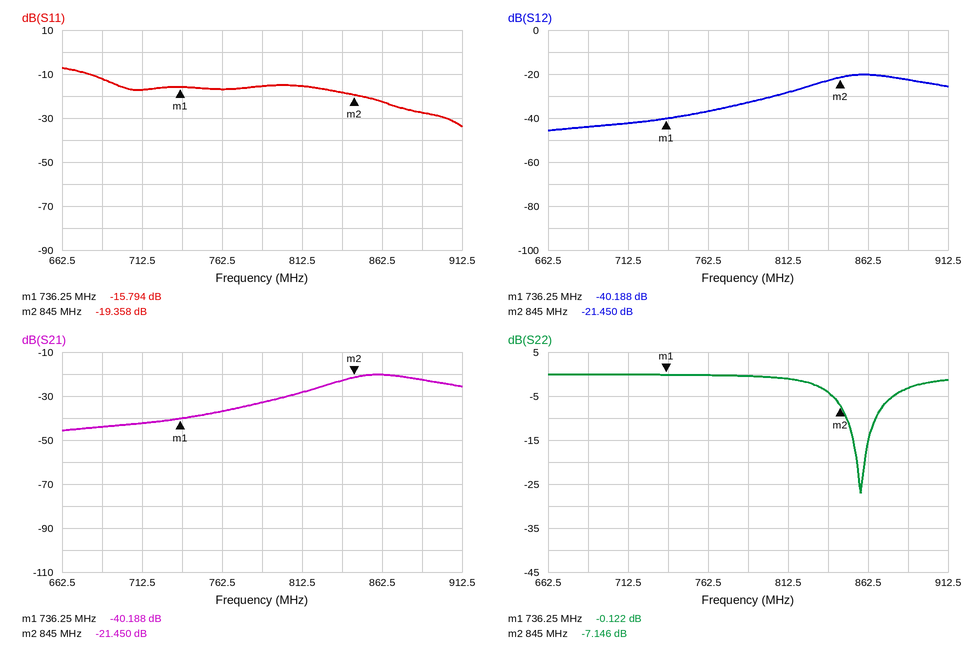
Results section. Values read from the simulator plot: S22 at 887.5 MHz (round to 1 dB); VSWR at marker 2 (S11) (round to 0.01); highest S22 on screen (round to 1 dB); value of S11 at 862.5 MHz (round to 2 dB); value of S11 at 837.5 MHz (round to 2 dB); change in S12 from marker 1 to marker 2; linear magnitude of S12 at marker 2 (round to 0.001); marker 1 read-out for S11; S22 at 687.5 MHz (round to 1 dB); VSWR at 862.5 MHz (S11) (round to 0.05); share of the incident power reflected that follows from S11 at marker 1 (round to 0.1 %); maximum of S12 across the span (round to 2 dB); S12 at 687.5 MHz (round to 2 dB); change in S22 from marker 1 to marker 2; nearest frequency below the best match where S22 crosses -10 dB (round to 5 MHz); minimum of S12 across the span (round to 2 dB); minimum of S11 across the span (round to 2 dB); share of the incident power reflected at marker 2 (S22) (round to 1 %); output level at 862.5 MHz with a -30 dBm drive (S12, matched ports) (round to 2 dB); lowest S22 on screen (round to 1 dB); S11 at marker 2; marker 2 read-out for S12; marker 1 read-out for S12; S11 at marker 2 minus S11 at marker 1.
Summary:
-3 dB
1.24
0 dB
-22 dB
-18 dB
18.738 dB
0.085
-15.794 dB
0 dB
1.15
2.6 %
-20 dB
-44 dB
-7.024 dB
850 MHz
-46 dB
-34 dB
19 %
-50 dBm
-27 dB
-19.358 dB
-21.450 dB
-40.188 dB
-3.564 dB
